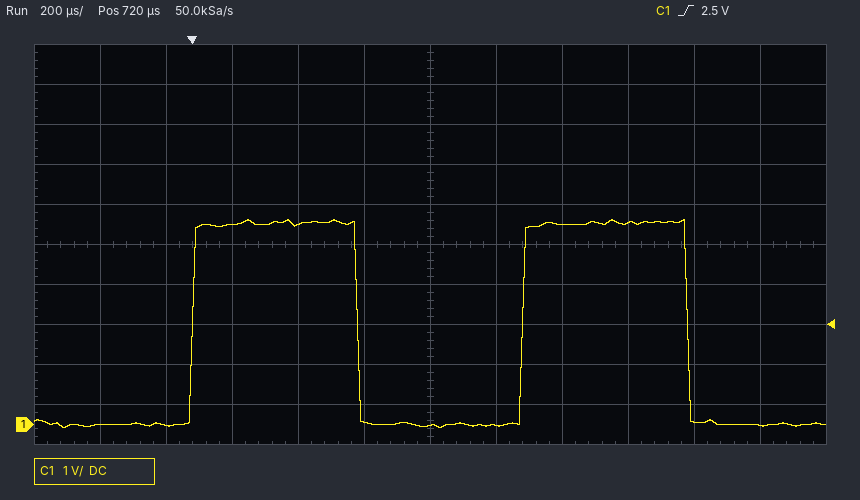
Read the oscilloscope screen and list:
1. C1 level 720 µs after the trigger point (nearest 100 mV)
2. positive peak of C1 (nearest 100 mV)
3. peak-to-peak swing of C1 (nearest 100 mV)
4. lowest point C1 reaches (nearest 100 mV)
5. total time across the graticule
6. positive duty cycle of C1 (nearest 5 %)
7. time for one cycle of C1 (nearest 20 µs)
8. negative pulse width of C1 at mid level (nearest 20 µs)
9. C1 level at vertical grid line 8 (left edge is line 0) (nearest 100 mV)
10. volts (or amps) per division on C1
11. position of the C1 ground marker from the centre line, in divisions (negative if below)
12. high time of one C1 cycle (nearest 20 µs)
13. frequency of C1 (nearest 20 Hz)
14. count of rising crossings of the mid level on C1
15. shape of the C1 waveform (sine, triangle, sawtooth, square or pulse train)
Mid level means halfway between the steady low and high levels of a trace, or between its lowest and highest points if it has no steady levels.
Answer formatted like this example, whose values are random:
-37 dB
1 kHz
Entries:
0.0 V
5.1 V
5.2 V
-100 mV
2.4 ms
50 %
1.00 ms
500 µs
5.0 V
1 V
-4.5 div
500 µs
1.00 kHz
2
square
